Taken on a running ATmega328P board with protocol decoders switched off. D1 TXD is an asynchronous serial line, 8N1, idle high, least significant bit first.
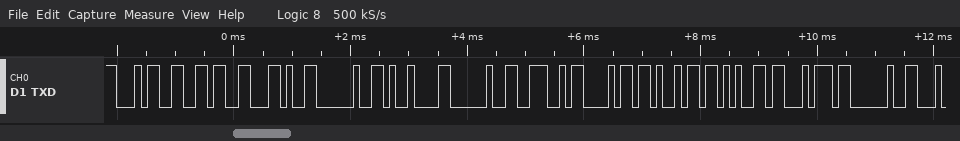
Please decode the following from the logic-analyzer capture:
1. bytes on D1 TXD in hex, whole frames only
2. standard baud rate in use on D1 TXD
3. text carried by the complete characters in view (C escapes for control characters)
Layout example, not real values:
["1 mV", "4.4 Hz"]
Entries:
["0x34 0x36 0x2C 0x20 0x09 0x20 0x4E 0x68 0x69 0x65 0x74 0x20", "9600 baud", "\"46, \\t Nhiet \""]
